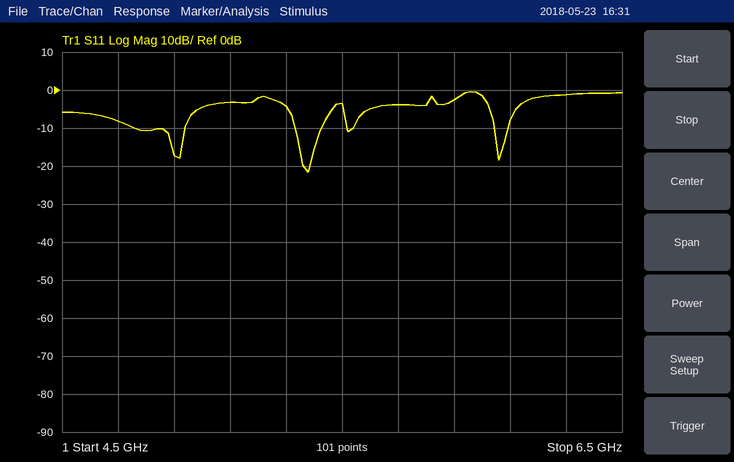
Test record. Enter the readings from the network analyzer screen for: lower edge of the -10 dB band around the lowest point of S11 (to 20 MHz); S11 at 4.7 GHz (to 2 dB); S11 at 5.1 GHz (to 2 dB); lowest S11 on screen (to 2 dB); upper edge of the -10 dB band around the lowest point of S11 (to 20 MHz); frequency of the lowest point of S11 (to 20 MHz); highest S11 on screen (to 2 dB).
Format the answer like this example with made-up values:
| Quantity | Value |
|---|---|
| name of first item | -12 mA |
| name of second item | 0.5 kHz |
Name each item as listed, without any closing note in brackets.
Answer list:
| Quantity | Value |
|---|---|
| lower edge of the -10 dB band around the lowest point of S11 | 5.34 GHz |
| S11 at 4.7 GHz | -8 dB |
| S11 at 5.1 GHz | -4 dB |
| lowest S11 on screen | -22 dB |
| upper edge of the -10 dB band around the lowest point of S11 | 5.42 GHz |
| frequency of the lowest point of S11 | 5.38 GHz |
| highest S11 on screen | 0 dB |
